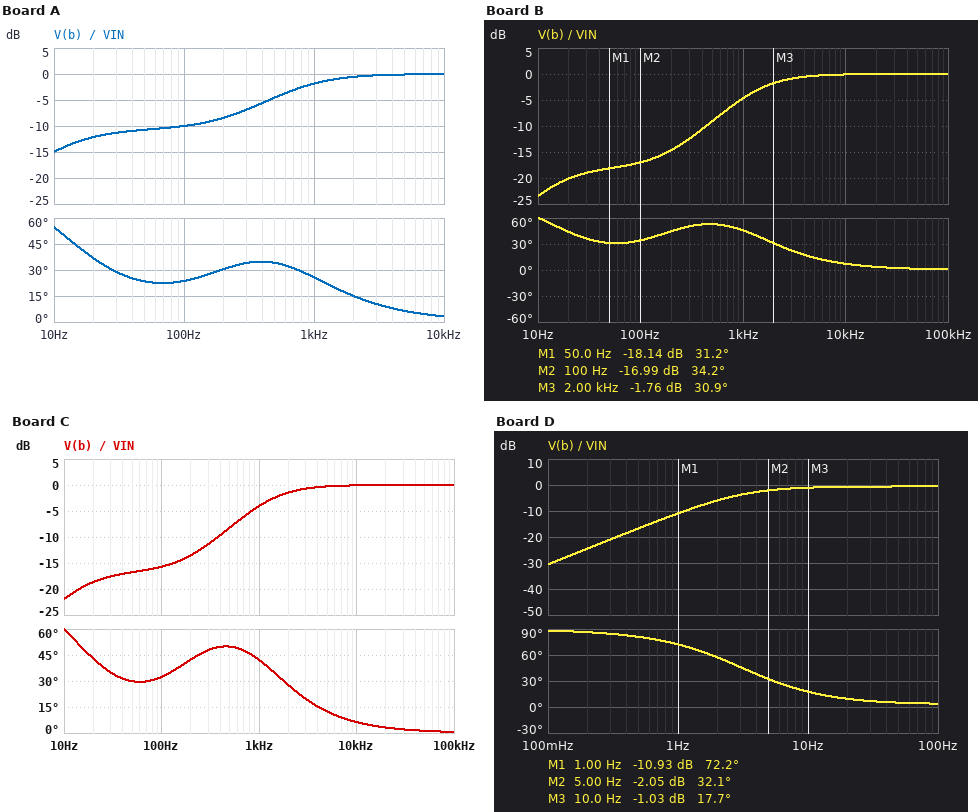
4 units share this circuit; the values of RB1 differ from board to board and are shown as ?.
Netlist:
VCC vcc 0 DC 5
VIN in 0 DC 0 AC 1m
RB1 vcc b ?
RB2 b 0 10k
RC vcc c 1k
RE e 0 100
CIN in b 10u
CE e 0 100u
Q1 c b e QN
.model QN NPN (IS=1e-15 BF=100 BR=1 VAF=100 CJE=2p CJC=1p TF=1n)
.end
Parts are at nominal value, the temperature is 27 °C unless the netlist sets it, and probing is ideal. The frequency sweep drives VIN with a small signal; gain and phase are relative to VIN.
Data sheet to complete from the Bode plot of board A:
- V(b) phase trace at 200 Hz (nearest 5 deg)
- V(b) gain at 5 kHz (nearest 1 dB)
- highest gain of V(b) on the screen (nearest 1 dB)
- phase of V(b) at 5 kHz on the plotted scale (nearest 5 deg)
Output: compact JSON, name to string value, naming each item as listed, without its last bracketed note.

{"V(b) phase trace at 200 Hz": "30 deg", "V(b) gain at 5 kHz": "0 dB", "highest gain of V(b) on the screen": "0 dB", "phase of V(b) at 5 kHz on the plotted scale": "5 deg"}
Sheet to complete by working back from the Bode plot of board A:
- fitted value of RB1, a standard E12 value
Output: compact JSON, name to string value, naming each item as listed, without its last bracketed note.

{"fitted value of RB1, a standard E12 value": "22 kΩ"}
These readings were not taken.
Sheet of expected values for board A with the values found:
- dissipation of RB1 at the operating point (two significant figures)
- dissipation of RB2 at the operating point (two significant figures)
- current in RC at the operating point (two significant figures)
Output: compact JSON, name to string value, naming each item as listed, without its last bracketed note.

{"dissipation of RB1 at the operating point": "660 µW", "dissipation of RB2 at the operating point": "140 µW", "current in RC at the operating point": "4.4 mA"}
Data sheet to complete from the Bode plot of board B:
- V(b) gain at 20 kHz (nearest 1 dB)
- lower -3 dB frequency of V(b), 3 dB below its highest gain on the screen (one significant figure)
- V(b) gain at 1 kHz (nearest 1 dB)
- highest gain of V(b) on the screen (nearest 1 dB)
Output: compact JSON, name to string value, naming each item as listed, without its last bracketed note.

{"V(b) gain at 20 kHz": "0 dB", "lower -3 dB frequency of V(b), 3 dB below its highest gain on the screen": "1 kHz", "V(b) gain at 1 kHz": "-5 dB", "highest gain of V(b) on the screen": "0 dB"}
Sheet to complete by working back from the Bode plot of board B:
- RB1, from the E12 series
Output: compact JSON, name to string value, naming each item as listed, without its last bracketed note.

{"RB1, from the E12 series": "15 kΩ"}
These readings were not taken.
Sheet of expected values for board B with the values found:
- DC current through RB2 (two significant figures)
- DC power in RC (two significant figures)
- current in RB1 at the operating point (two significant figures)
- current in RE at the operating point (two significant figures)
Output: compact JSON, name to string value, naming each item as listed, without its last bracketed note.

{"DC current through RB2": "120 µA", "DC power in RC": "20 mW", "current in RB1 at the operating point": "250 µA", "current in RE at the operating point": "4.6 mA"}
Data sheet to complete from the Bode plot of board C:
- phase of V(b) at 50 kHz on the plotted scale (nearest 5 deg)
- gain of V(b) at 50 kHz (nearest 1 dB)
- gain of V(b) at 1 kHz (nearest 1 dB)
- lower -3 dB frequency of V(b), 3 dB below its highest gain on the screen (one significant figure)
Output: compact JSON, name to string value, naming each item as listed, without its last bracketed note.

{"phase of V(b) at 50 kHz on the plotted scale": "0 deg", "gain of V(b) at 50 kHz": "0 dB", "gain of V(b) at 1 kHz": "-4 dB", "lower -3 dB frequency of V(b), 3 dB below its highest gain on the screen": "1 kHz"}
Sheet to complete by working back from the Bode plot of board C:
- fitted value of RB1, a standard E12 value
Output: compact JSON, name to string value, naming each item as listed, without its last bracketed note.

{"fitted value of RB1, a standard E12 value": "18 kΩ"}
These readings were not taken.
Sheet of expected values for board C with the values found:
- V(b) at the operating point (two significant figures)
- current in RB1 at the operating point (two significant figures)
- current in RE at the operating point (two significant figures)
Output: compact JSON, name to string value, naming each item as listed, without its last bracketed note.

{"V(b) at the operating point": "1.2 V", "current in RB1 at the operating point": "210 µA", "current in RE at the operating point": "4.5 mA"}
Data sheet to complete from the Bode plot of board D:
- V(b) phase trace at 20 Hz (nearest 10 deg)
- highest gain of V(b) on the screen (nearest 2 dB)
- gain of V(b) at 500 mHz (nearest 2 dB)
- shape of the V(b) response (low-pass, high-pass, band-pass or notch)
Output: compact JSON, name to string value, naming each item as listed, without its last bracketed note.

{"V(b) phase trace at 20 Hz": "10 deg", "highest gain of V(b) on the screen": "0 dB", "gain of V(b) at 500 mHz": "-16 dB", "shape of the V(b) response": "high-pass"}
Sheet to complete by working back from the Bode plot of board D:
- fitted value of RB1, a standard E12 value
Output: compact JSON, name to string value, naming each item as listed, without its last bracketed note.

{"fitted value of RB1, a standard E12 value": "39 kΩ"}
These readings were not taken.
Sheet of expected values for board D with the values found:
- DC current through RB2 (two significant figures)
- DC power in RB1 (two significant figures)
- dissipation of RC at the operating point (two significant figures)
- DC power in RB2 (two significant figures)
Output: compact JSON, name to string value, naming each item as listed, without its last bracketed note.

{"DC current through RB2": "89 µA", "DC power in RB1": "430 µW", "dissipation of RC at the operating point": "2.7 mW", "DC power in RB2": "80 µW"}
